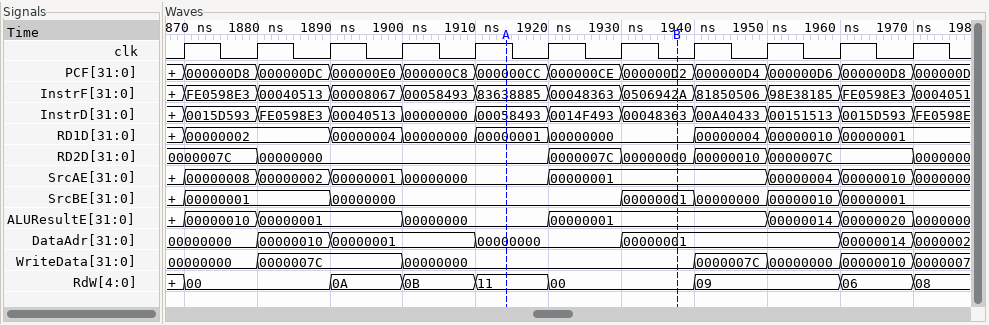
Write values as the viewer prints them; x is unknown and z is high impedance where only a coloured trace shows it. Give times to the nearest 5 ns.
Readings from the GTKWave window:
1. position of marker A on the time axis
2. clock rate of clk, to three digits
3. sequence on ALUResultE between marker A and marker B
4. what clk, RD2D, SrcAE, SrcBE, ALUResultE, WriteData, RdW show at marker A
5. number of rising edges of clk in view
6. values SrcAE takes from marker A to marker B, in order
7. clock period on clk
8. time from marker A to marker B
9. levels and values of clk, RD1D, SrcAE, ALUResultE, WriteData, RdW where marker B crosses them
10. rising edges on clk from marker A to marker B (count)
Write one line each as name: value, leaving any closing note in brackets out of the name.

position of marker A on the time axis: 1915 ns
clock rate of clk, to three digits: 100 MHz
sequence on ALUResultE between marker A and marker B: 00000000, 00000001
what clk, RD2D, SrcAE, SrcBE, ALUResultE, WriteData, RdW show at marker A: clk=1, RD2D=00000000, SrcAE=00000000, SrcBE=00000000, ALUResultE=00000000, WriteData=00000000, RdW=11
number of rising edges of clk in view: 11
values SrcAE takes from marker A to marker B, in order: 00000000, 00000001
clock period on clk: 10 ns
time from marker A to marker B: 25 ns
levels and values of clk, RD1D, SrcAE, ALUResultE, WriteData, RdW where marker B crosses them: clk=0, RD1D=00000000, SrcAE=00000001, ALUResultE=00000001, WriteData=00000000, RdW=00
rising edges on clk from marker A to marker B: 2
